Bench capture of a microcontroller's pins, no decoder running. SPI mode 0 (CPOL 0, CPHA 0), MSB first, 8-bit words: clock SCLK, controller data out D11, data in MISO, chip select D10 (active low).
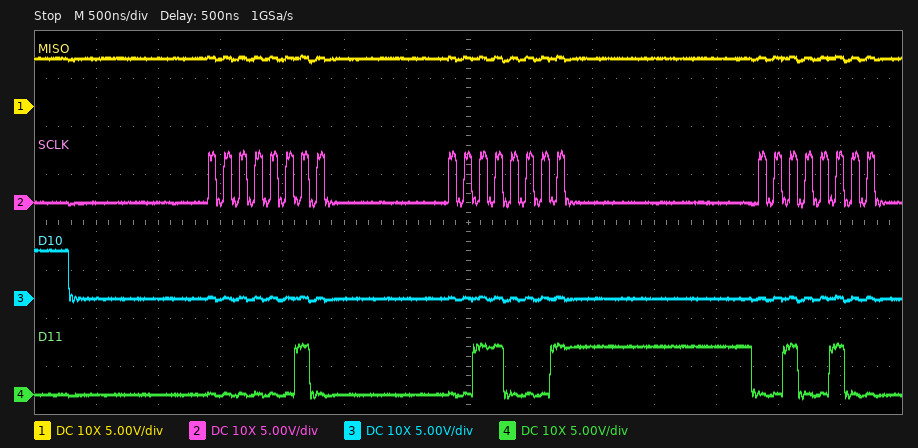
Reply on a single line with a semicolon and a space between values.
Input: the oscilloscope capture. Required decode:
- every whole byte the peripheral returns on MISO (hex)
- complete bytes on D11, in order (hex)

0xFF 0xFF 0xFF; 0x02 0x31 0x24
